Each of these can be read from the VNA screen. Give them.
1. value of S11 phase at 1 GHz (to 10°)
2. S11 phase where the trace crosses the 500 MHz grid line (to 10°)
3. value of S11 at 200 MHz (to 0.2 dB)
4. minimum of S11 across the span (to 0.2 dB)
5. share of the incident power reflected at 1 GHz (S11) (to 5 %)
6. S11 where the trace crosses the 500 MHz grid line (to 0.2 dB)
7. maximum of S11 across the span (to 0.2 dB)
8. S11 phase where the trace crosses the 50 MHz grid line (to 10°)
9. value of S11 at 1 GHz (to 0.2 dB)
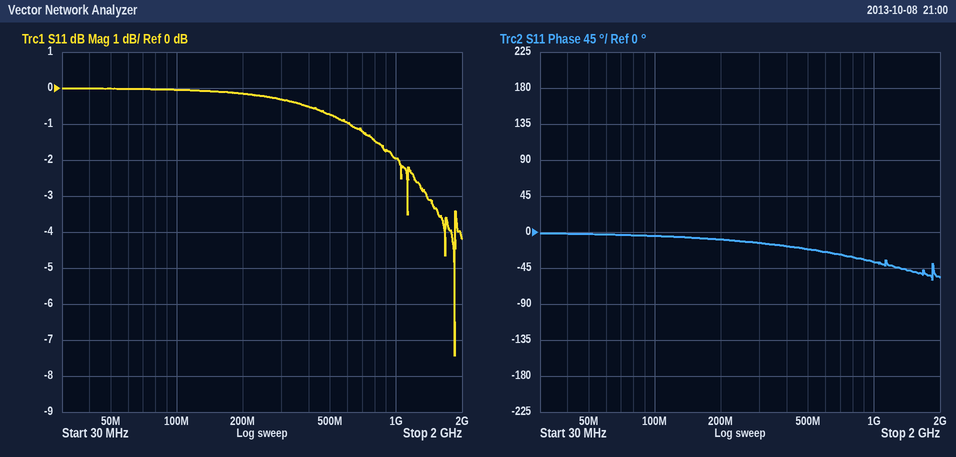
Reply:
-40°
-20°
-0.2 dB
-7.4 dB
65 %
-0.8 dB
0.0 dB
0°
-2.0 dB
